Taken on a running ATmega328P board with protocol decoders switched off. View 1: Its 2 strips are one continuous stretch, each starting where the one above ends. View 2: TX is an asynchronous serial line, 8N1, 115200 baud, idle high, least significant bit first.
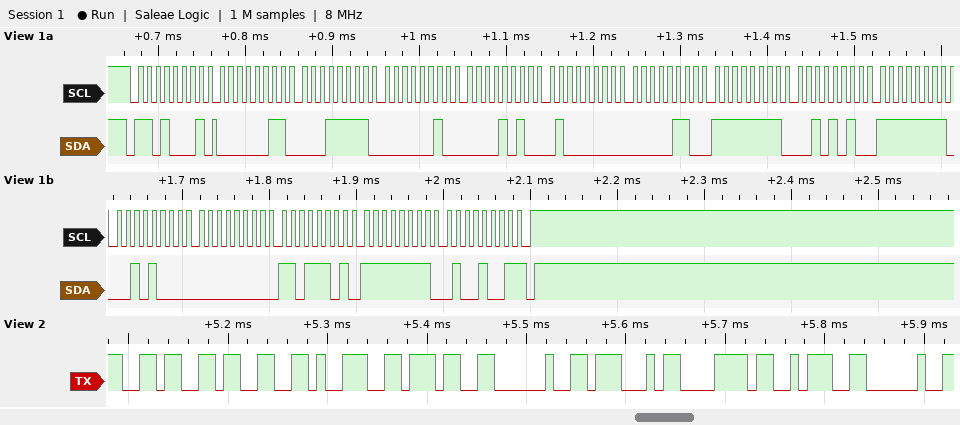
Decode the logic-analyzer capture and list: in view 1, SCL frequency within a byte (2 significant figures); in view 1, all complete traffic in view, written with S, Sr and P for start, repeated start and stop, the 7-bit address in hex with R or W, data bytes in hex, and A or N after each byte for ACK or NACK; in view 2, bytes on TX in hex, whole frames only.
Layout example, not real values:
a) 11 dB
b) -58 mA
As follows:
a) 100 kHz
b) S 68R A 03 A 1F A 02 A 0A A 40 A 06 A FF A 2A A FF A 28 A 00 A DD A FF A 49 N P
c) 36 33 39 37 20 47 78 3A 20
